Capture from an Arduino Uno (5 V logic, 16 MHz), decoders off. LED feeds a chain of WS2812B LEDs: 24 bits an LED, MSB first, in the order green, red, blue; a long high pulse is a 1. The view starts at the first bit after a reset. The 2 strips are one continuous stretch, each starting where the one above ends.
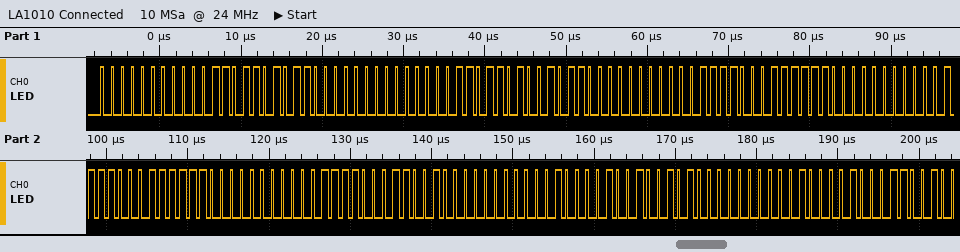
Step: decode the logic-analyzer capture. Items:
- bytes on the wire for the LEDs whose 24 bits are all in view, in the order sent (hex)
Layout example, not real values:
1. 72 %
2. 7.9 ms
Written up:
1. 00 1B 58 00 1B 4B 00 1E 3F 00 1E 3F 00 1E 32 00 21 25 00 21 19
